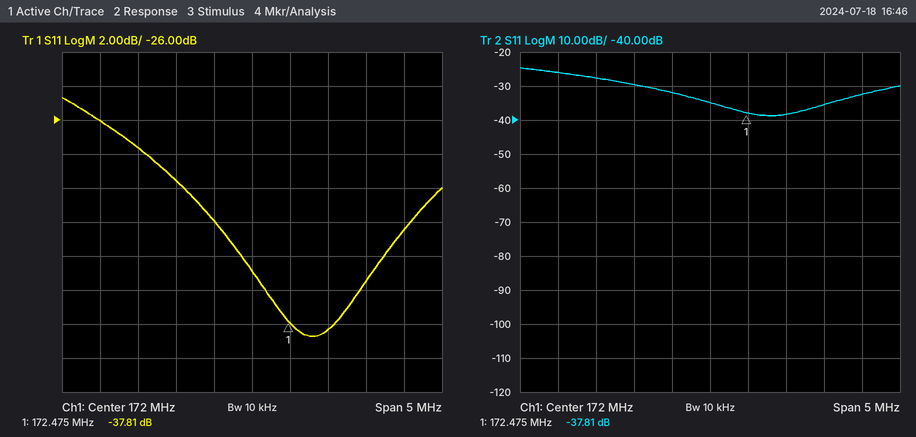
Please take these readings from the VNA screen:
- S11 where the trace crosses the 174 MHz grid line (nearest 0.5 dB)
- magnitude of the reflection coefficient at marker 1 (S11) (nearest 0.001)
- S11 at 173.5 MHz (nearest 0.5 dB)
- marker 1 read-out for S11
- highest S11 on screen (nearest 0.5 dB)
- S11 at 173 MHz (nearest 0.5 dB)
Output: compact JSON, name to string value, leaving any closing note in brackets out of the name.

{"S11 where the trace crosses the 174 MHz grid line": "-32.5 dB", "magnitude of the reflection coefficient at marker 1 (S11)": "0.013", "S11 at 173.5 MHz": "-35.5 dB", "marker 1 read-out for S11": "-37.81 dB", "highest S11 on screen": "-24.5 dB", "S11 at 173 MHz": "-38.5 dB"}
